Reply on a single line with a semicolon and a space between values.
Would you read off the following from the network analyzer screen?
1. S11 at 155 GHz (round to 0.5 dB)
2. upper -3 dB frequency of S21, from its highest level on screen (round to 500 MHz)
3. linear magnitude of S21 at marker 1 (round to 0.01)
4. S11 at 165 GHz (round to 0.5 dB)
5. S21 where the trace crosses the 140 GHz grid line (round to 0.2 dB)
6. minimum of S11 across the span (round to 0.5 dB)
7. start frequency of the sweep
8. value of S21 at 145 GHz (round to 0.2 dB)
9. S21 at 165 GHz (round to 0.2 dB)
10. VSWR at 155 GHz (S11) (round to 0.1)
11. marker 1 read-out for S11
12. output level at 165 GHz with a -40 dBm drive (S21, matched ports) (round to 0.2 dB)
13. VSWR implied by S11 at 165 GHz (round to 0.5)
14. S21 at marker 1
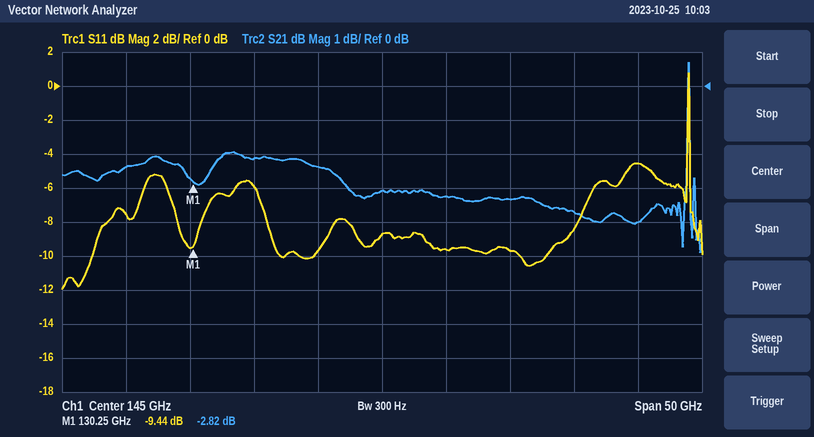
-9.5 dB; 169.0 GHz; 0.72; -4.5 dB; -2.4 dB; -12.0 dB; 120 GHz; -3.0 dB; -4.0 dB; 2.0; -9.44 dB; -44.0 dBm; 4.0; -2.82 dB
